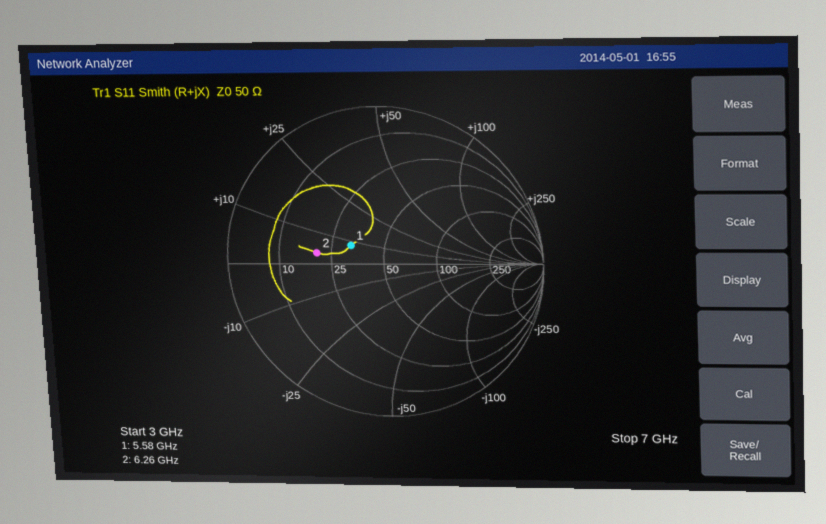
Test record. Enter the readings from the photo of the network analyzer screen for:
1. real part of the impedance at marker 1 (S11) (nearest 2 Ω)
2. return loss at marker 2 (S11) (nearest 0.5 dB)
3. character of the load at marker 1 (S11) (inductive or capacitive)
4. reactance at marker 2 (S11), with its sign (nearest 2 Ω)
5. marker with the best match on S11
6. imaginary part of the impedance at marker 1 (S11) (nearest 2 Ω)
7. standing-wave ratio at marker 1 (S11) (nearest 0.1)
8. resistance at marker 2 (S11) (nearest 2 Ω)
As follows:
32 Ω
7.5 dB
inductive
+4 Ω
marker 1
+8 Ω
1.6
20 Ω
